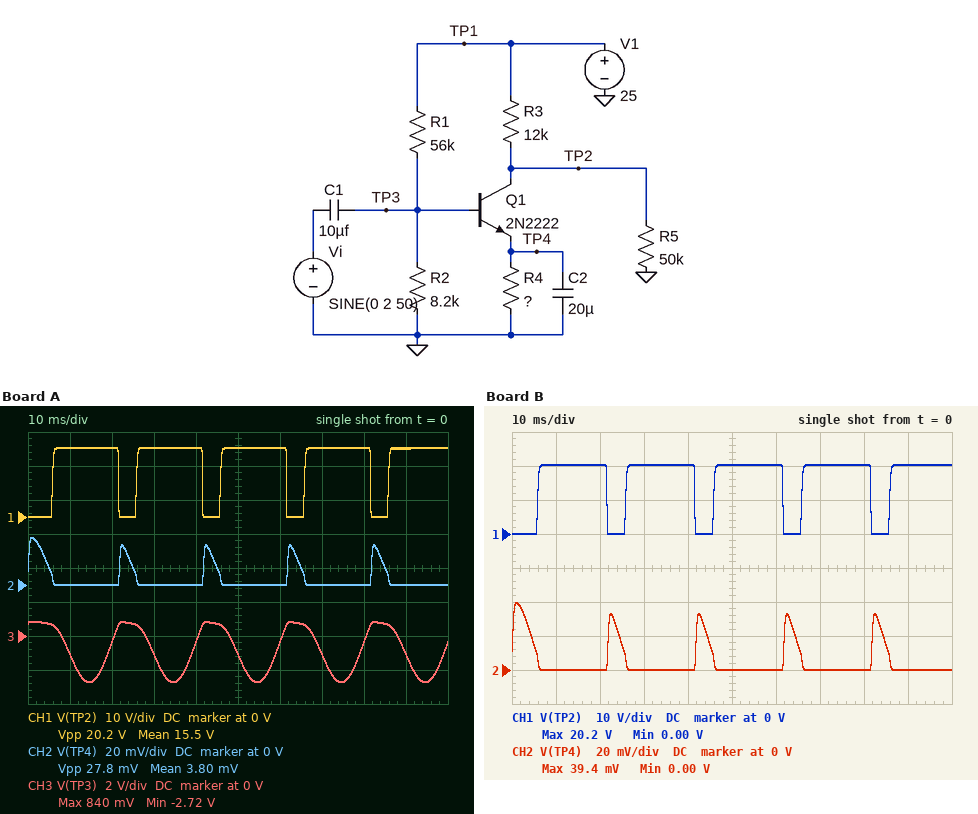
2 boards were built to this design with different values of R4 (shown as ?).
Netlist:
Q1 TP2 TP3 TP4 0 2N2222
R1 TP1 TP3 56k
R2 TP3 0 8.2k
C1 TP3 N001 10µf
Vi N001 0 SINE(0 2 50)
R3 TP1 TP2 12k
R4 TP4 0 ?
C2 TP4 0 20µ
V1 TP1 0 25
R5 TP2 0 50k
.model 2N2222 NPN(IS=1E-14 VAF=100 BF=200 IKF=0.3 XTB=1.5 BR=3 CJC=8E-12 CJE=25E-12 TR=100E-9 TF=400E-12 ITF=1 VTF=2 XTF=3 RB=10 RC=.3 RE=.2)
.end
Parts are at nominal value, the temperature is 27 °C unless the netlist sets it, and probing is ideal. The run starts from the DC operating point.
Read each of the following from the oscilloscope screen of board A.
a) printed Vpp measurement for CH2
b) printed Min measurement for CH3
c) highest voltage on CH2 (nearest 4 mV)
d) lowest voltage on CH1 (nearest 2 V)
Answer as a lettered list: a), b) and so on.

a) 27.8 mV
b) -2.72 V
c) 28 mV
d) 0 V
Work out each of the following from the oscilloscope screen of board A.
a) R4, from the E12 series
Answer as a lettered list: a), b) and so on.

a) 3.3 Ω
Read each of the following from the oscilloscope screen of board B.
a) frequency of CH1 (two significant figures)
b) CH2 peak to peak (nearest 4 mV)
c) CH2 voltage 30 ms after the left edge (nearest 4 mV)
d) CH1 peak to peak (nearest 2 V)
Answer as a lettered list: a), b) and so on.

a) 50 Hz
b) 40 mV
c) 0 V
d) 20 V
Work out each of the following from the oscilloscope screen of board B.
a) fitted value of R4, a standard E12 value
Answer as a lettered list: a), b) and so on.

a) 4.7 Ω
